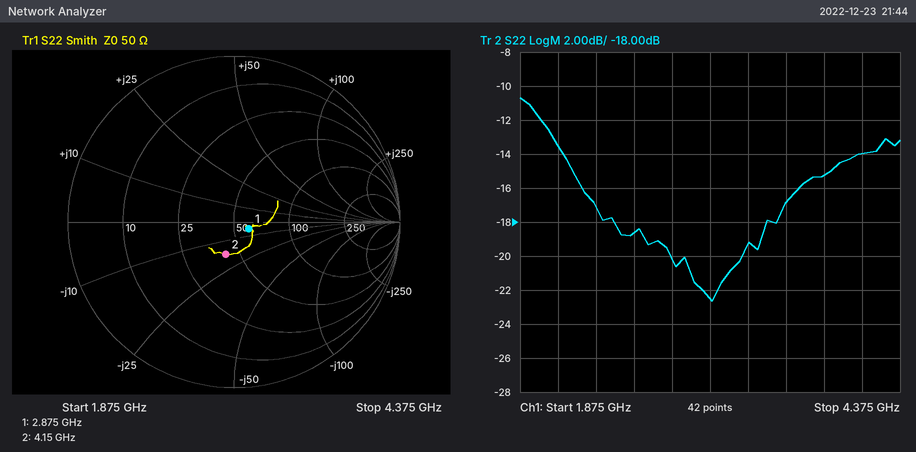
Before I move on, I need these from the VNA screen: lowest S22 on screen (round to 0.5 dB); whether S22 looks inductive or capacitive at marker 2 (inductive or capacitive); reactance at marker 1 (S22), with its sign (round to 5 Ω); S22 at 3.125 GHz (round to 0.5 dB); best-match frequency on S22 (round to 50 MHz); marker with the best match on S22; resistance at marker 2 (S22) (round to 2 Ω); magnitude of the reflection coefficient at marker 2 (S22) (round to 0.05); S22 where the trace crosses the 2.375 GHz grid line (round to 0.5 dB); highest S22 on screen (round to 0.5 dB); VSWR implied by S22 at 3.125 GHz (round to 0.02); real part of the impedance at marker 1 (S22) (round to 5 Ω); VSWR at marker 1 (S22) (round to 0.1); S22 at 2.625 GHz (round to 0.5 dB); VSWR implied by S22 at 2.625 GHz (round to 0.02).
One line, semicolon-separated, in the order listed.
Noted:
-22.5 dB; capacitive; -5 Ω; -22.5 dB; 3.15 GHz; marker 1; 42 Ω; 0.20; -17.0 dB; -10.5 dB; 1.16; 60 Ω; 1.2; -18.5 dB; 1.26
